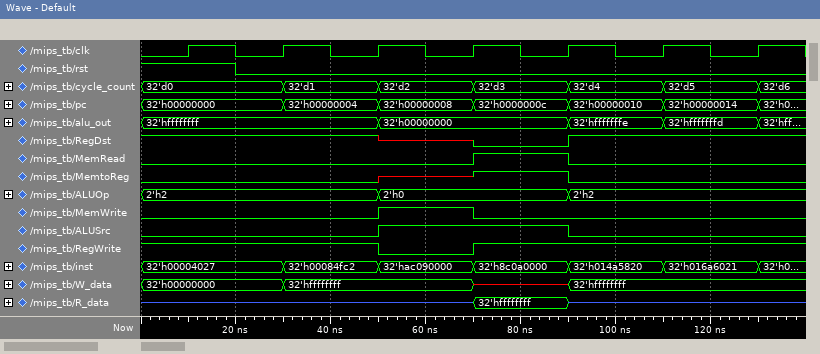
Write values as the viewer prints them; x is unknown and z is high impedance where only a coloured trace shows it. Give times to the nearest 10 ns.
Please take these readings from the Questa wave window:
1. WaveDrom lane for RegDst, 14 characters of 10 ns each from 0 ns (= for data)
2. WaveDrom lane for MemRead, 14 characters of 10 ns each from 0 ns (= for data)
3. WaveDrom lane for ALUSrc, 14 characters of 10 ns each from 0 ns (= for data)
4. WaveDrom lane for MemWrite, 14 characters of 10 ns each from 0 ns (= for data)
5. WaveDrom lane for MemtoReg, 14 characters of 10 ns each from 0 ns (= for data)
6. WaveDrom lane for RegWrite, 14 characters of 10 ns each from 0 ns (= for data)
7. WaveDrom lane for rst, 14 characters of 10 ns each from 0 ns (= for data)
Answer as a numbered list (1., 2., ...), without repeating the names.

1. {name: 'RegDst', wave: '1....x.0.1....'}
2. {name: 'MemRead', wave: '0......1.0....'}
3. {name: 'ALUSrc', wave: '0....1...0....'}
4. {name: 'MemWrite', wave: '0....1.0......'}
5. {name: 'MemtoReg', wave: '0....x.1.0....'}
6. {name: 'RegWrite', wave: '1....0.1......'}
7. {name: 'rst', wave: '1.0...........'}
